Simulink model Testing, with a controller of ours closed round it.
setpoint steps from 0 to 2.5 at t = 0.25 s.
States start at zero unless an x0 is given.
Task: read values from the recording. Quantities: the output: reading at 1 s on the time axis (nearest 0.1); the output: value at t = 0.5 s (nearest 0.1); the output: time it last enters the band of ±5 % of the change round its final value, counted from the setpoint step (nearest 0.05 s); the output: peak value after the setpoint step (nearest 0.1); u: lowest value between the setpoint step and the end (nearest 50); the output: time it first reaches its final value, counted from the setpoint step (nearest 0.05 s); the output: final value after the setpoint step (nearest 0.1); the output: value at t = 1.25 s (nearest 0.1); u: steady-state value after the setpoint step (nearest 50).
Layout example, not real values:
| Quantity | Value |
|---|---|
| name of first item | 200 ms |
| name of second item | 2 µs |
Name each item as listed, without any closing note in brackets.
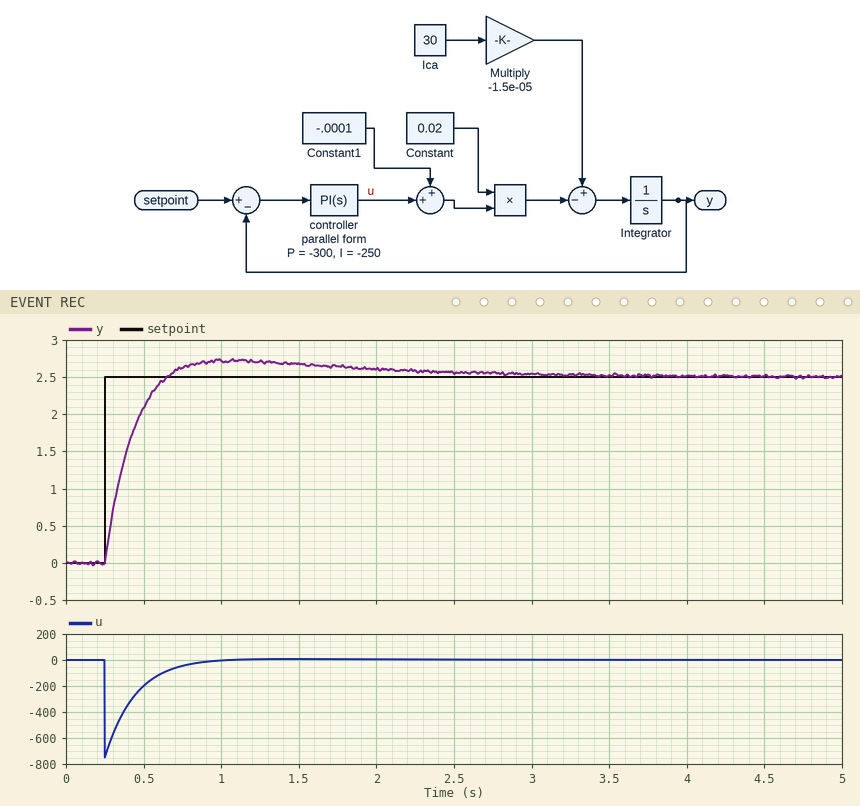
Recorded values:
| Quantity | Value |
|---|---|
| the output: reading at 1 s on the time axis | 2.7 |
| the output: value at t = 0.5 s | 2.1 |
| the output: time it last enters the band of ±5 % of the change round its final value, counted from the setpoint step | 1.60 s |
| the output: peak value after the setpoint step | 2.7 |
| u: lowest value between the setpoint step and the end | -750 |
| the output: time it first reaches its final value, counted from the setpoint step | 0.40 s |
| the output: final value after the setpoint step | 2.5 |
| the output: value at t = 1.25 s | 2.7 |
| u: steady-state value after the setpoint step | 0 |
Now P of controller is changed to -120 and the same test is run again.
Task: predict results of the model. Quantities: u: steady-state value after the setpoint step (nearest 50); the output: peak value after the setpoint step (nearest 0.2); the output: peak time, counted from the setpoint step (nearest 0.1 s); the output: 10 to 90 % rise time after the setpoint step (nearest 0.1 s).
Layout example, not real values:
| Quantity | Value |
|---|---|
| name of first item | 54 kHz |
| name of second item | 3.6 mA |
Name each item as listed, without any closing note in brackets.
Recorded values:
| Quantity | Value |
|---|---|
| u: steady-state value after the setpoint step | 0 |
| the output: peak value after the setpoint step | 3.2 |
| the output: peak time, counted from the setpoint step | 1.1 s |
| the output: 10 to 90 % rise time after the setpoint step | 0.4 s |
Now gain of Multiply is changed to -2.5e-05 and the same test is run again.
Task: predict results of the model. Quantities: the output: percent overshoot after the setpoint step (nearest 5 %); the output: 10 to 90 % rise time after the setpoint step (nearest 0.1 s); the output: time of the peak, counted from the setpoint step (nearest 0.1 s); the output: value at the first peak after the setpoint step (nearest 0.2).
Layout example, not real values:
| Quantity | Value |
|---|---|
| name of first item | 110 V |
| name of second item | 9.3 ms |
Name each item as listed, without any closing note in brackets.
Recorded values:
| Quantity | Value |
|---|---|
| the output: percent overshoot after the setpoint step | 10 % |
| the output: 10 to 90 % rise time after the setpoint step | 0.3 s |
| the output: time of the peak, counted from the setpoint step | 0.8 s |
| the output: value at the first peak after the setpoint step | 2.8 |
